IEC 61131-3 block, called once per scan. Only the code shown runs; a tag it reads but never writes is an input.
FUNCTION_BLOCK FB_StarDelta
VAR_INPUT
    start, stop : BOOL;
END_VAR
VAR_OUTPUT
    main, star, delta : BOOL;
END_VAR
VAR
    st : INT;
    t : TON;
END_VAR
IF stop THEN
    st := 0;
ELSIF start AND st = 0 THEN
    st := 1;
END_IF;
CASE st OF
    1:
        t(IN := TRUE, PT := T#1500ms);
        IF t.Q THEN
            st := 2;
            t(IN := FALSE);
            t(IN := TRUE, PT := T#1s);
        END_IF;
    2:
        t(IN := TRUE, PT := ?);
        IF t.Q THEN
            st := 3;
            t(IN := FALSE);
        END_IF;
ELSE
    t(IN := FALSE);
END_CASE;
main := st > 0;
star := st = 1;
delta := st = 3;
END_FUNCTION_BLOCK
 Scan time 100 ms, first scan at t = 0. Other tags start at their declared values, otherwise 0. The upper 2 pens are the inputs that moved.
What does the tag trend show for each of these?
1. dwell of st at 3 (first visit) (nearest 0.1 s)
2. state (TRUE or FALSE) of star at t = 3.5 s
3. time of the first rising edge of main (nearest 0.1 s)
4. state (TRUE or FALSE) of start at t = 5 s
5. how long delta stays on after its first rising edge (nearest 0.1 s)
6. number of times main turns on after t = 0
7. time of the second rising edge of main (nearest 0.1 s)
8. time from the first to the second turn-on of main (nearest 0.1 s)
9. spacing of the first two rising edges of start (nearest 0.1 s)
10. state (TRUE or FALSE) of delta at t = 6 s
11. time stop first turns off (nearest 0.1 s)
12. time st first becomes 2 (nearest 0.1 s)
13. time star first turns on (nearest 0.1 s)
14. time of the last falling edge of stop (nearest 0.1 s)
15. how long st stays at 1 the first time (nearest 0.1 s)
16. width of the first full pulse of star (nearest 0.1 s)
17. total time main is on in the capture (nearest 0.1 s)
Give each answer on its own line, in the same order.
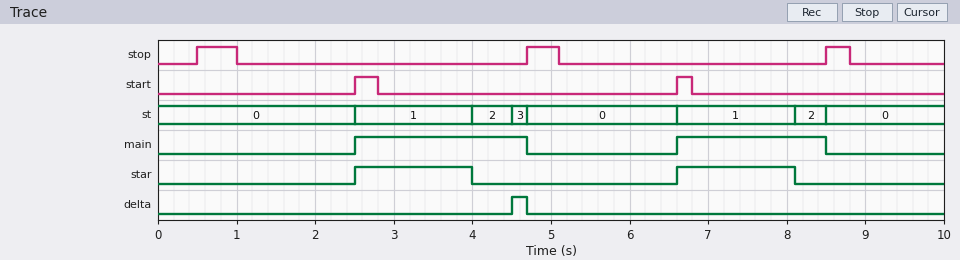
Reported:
0.2 s
TRUE
2.5 s
FALSE
0.2 s
2
6.6 s
4.1 s
4.1 s
FALSE
1.0 s
4.0 s
2.5 s
8.8 s
1.5 s
1.5 s
4.1 s
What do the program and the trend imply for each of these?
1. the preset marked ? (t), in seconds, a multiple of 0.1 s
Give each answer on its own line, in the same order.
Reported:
0.5 s
